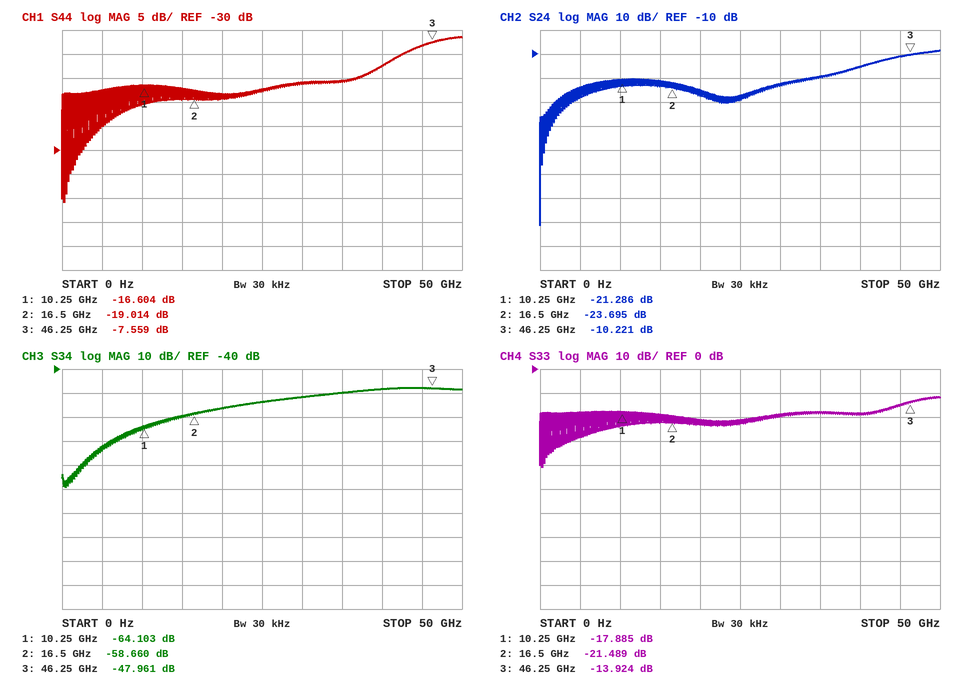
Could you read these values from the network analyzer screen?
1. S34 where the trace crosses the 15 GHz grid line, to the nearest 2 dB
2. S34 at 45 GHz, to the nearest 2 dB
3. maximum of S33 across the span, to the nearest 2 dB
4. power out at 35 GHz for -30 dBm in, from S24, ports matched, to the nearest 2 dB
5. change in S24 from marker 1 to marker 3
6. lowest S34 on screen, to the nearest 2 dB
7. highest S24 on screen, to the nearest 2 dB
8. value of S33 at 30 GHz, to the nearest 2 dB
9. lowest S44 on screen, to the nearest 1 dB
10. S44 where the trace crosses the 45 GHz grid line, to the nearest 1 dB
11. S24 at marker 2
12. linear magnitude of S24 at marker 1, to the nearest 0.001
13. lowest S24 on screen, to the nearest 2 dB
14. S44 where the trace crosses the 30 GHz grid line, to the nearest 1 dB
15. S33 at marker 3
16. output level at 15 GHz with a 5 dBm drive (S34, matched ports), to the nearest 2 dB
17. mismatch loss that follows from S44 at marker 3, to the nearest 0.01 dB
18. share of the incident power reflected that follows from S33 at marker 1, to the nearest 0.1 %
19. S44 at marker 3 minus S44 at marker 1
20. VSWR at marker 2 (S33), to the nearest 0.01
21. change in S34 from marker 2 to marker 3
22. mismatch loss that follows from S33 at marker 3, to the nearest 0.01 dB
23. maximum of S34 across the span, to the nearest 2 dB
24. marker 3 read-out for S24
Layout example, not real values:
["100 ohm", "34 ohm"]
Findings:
["-60 dB", "-48 dB", "-12 dB", "-50 dBm", "11.065 dB", "-90 dB", "-8 dB", "-20 dB", "-41 dB", "-8 dB", "-23.695 dB", "0.086", "-82 dB", "-16 dB", "-13.924 dB", "-54 dBm", "0.84 dB", "1.6 %", "9.045 dB", "1.18", "10.699 dB", "0.18 dB", "-48 dB", "-10.221 dB"]
